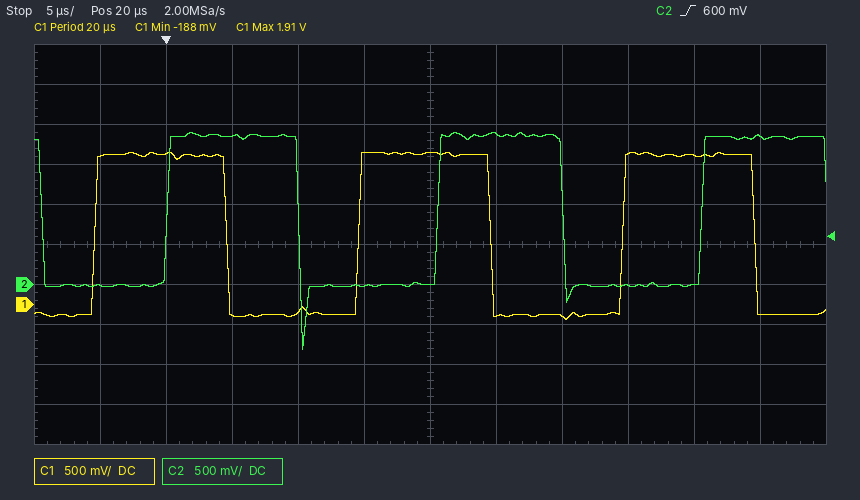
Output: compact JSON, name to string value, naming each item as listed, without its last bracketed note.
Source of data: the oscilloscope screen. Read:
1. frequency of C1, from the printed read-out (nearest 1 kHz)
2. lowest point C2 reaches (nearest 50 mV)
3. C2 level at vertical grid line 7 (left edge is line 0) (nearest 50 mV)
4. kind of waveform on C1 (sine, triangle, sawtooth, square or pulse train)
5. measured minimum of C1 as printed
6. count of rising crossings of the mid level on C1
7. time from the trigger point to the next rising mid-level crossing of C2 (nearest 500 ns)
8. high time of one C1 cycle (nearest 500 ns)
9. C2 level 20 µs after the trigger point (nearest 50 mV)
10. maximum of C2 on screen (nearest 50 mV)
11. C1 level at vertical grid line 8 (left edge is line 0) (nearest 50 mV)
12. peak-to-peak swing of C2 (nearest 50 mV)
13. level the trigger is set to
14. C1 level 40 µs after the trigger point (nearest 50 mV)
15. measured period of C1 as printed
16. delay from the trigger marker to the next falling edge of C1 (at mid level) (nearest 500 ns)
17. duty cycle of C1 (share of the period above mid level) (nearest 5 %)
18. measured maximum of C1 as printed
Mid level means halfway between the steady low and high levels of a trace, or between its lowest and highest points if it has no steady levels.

{"frequency of C1, from the printed read-out": "50 kHz", "lowest point C2 reaches": "-800 mV", "C2 level at vertical grid line 7 (left edge is line 0)": "1.90 V", "kind of waveform on C1": "square", "measured minimum of C1 as printed": "-188 mV", "count of rising crossings of the mid level on C1": "3", "time from the trigger point to the next rising mid-level crossing of C2": "20.5 µs", "high time of one C1 cycle": "10.0 µs", "C2 level 20 µs after the trigger point": "0 mV", "maximum of C2 on screen": "1.90 V", "C1 level at vertical grid line 8 (left edge is line 0)": "-150 mV", "peak-to-peak swing of C2": "2.70 V", "level the trigger is set to": "600 mV", "C1 level 40 µs after the trigger point": "1.85 V", "measured period of C1 as printed": "20 µs", "delay from the trigger marker to the next falling edge of C1 (at mid level)": "4.5 µs", "duty cycle of C1 (share of the period above mid level)": "50 %", "measured maximum of C1 as printed": "1.91 V"}
